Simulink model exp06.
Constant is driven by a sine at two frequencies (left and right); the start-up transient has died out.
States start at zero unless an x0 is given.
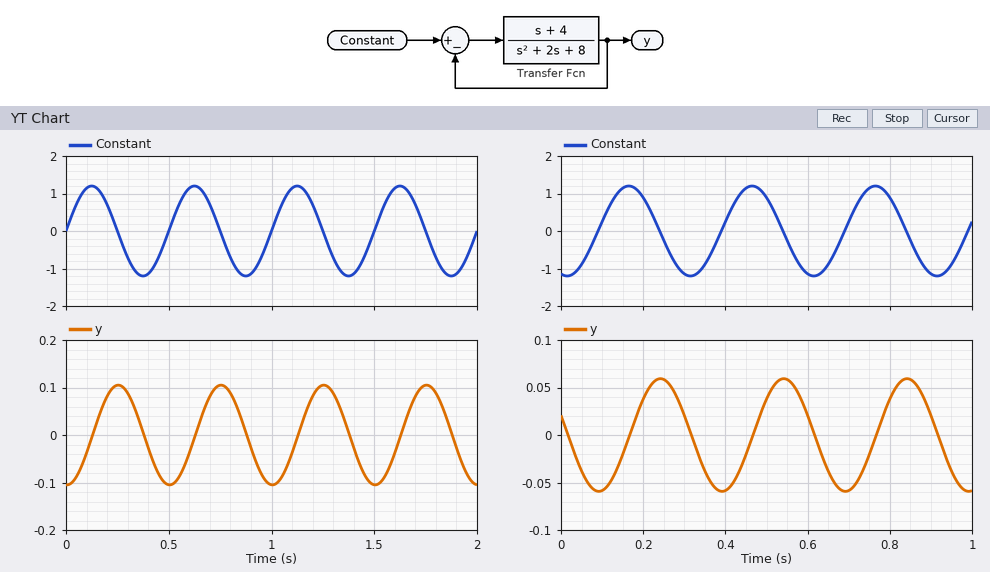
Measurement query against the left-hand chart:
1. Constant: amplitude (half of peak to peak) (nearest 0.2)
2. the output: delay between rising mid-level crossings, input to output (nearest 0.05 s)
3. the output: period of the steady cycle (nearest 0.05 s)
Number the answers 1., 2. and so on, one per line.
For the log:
1. 1.2
2. 0.15 s
3. 0.50 s
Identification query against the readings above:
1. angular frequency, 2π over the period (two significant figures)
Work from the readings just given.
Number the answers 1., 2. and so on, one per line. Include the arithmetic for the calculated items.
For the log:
1. 2π / 0.5 = 13 rad/s
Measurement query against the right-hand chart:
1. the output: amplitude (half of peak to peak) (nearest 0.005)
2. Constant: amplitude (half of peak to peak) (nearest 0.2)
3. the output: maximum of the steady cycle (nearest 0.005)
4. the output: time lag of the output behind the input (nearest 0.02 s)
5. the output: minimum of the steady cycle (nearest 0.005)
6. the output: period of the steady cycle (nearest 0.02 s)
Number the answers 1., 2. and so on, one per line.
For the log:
1. 0.060
2. 1.2
3. 0.060
4. 0.08 s
5. -0.060
6. 0.30 s
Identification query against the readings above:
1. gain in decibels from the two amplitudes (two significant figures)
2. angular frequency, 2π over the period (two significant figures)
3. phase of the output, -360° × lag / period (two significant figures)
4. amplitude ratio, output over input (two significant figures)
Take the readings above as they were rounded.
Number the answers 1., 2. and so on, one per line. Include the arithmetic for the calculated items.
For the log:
1. 20 log10(0.06 / 1.2) = -26 dB
2. 2π / 0.3 = 21 rad/s
3. -360 × 0.08 / 0.3 = -96°
4. 0.06 / 1.2 = 0.050
